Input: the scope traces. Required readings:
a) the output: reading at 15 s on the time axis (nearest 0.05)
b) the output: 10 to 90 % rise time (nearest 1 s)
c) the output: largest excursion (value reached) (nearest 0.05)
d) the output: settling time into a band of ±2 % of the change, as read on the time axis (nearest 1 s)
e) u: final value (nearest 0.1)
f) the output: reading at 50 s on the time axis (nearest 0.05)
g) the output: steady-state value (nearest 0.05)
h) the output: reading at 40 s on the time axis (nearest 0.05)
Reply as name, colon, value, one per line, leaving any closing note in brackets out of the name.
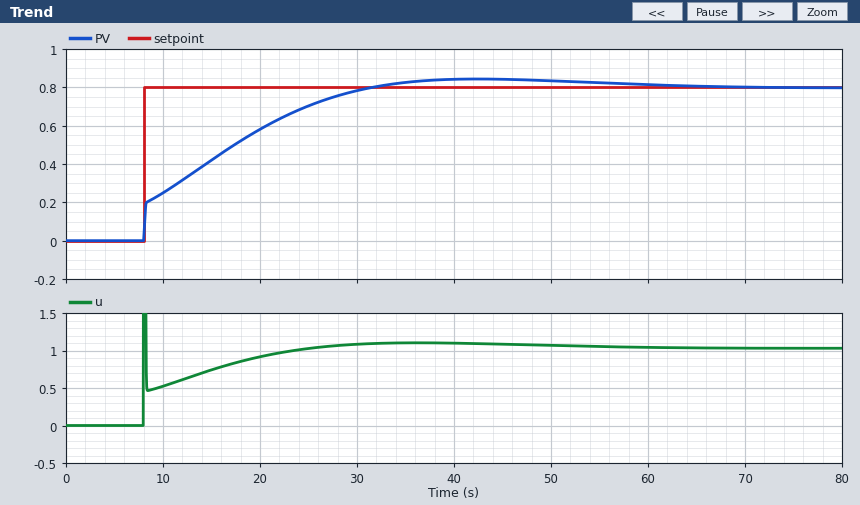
the output: reading at 15 s on the time axis: 0.40
the output: 10 to 90 % rise time: 18 s
the output: largest excursion (value reached): 0.85
the output: settling time into a band of ±2 % of the change, as read on the time axis: 59 s
u: final value: 1.0
the output: reading at 50 s on the time axis: 0.85
the output: steady-state value: 0.80
the output: reading at 40 s on the time axis: 0.85
